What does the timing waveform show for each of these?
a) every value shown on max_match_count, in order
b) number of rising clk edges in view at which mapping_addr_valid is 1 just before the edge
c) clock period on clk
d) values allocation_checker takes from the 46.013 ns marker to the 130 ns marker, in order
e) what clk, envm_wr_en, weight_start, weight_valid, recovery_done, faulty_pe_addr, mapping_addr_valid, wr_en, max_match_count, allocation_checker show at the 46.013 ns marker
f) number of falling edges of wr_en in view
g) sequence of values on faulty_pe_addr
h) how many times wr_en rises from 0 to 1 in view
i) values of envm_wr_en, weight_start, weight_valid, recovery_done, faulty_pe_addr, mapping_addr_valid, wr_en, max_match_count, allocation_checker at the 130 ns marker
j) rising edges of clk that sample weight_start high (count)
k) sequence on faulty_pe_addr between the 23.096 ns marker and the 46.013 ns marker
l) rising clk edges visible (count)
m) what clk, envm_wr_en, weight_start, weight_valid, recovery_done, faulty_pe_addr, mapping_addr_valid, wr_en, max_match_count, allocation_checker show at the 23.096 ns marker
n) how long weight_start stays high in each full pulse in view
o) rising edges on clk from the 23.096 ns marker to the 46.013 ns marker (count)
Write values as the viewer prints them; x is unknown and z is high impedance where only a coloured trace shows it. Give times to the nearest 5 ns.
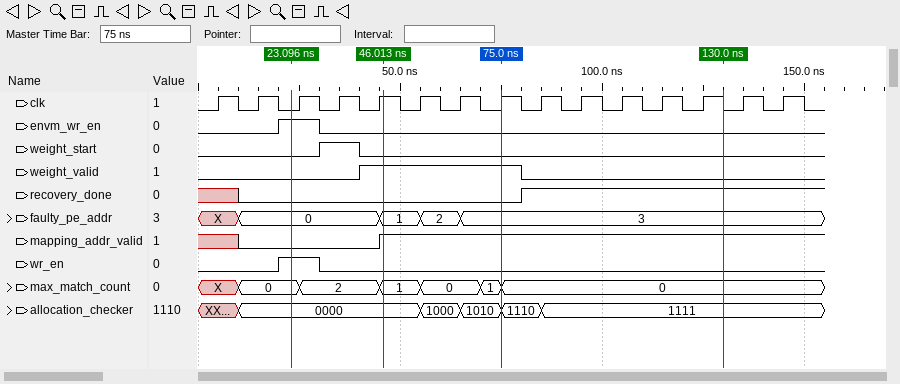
X, 0, 2, 1, 0, 1, 0
10
10 ns
0000, 1000, 1010, 1110, 1111
clk=1, envm_wr_en=0, weight_start=0, weight_valid=1, recovery_done=0, faulty_pe_addr=1, mapping_addr_valid=1, wr_en=0, max_match_count=1, allocation_checker=0000
1
X, 0, 1, 2, 3
1
envm_wr_en=0, weight_start=0, weight_valid=0, recovery_done=1, faulty_pe_addr=3, mapping_addr_valid=1, wr_en=0, max_match_count=0, allocation_checker=1111
1
0, 1
15
clk=0, envm_wr_en=1, weight_start=0, weight_valid=0, recovery_done=0, faulty_pe_addr=0, mapping_addr_valid=0, wr_en=1, max_match_count=0, allocation_checker=0000
10 ns
3
